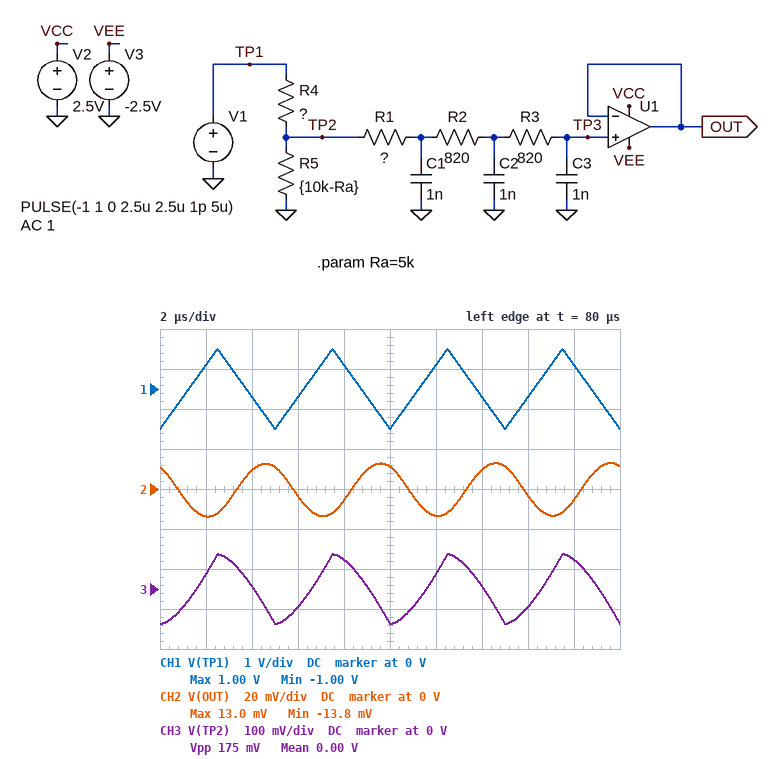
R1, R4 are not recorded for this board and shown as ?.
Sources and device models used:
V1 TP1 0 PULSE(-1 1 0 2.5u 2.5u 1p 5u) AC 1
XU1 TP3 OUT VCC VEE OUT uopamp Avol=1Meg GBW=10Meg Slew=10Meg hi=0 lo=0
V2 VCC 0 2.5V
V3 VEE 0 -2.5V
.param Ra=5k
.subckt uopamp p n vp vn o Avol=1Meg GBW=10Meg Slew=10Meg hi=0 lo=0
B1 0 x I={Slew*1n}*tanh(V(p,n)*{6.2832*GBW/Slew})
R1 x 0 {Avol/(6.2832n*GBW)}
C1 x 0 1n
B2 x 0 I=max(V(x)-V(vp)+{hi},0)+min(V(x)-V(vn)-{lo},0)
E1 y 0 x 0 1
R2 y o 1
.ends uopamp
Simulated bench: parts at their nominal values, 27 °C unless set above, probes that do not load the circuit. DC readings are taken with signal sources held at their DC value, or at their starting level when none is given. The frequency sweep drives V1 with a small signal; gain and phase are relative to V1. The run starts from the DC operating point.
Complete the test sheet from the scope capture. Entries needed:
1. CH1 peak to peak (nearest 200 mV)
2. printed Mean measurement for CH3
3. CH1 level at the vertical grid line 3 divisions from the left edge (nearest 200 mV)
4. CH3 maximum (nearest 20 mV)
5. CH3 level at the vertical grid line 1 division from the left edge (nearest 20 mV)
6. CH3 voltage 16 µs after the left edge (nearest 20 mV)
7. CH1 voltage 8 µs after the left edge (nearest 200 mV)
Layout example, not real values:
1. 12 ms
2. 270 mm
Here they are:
1. 2.0 V
2. 0.00 V
3. -200 mV
4. 80 mV
5. 40 mV
6. -40 mV
7. 600 mV
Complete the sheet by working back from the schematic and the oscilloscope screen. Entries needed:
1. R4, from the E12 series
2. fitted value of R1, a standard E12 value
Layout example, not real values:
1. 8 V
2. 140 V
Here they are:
1. 8.2 kΩ
2. 680 Ω
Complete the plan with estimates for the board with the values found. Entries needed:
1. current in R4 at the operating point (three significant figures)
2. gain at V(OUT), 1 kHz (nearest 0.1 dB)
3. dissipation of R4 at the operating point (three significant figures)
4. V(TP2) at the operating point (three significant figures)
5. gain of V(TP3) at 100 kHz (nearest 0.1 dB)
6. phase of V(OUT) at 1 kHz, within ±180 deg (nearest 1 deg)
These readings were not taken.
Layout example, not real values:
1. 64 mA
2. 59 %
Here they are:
1. 75.8 µA
2. -8.5 dB
3. 47.1 µW
4. -379 mV
5. -27.6 dB
6. -5 deg
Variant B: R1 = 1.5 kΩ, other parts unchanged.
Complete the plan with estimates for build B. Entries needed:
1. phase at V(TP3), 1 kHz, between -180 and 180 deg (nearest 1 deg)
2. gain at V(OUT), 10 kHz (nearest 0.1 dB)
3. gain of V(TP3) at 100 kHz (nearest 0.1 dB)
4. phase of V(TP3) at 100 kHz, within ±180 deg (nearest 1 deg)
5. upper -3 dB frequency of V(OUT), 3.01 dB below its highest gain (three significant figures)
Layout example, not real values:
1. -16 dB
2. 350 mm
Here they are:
1. -6 deg
2. -11.3 dB
3. -29.1 dB
4. -119 deg
5. 10.4 kHz
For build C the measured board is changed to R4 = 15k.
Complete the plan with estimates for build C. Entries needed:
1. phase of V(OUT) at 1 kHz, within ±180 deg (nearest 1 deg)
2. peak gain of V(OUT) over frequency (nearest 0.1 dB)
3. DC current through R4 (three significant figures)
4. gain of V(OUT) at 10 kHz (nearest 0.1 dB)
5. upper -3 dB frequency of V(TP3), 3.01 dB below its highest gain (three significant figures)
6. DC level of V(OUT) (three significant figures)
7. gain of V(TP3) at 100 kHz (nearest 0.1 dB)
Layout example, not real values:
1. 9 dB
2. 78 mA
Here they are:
1. -6 deg
2. -12.0 dB
3. 50.0 µA
4. -14.7 dB
5. 10.8 kHz
6. -250 mV
7. -32.4 dB
